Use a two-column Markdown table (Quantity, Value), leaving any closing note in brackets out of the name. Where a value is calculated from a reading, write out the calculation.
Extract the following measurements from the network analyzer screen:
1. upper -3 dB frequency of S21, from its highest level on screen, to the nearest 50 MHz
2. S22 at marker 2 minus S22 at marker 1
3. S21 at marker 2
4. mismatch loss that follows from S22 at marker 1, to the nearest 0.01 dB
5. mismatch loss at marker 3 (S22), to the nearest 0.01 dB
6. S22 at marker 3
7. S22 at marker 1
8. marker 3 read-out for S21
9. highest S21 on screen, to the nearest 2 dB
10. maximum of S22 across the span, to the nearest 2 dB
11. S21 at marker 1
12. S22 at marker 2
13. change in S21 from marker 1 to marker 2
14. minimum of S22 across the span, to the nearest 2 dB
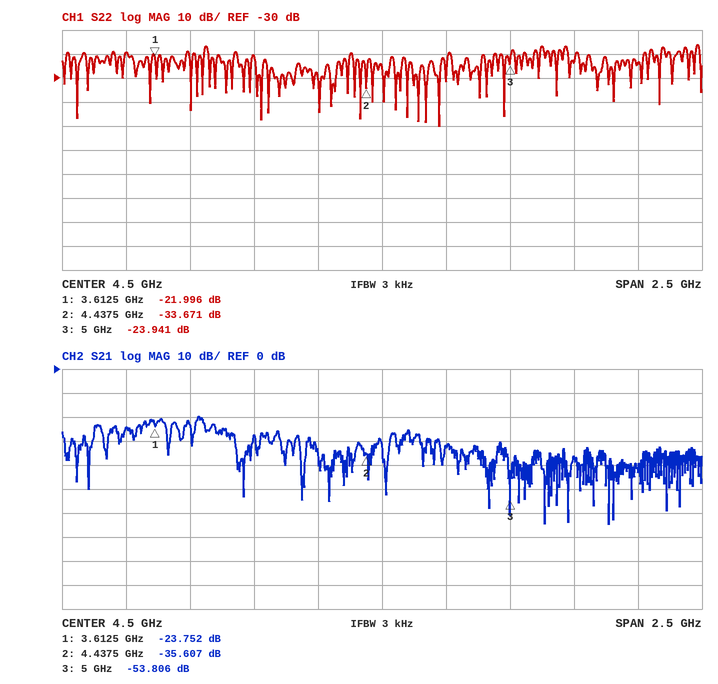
| Quantity | Value |
|---|---|
| upper -3 dB frequency of S21, from its highest level on screen, to the nearest 50 MHz | 3.80 GHz |
| S22 at marker 2 minus S22 at marker 1 | -33.671 − (-21.996) = -11.675 dB |
| S21 at marker 2 | -35.607 dB |
| mismatch loss that follows from S22 at marker 1, to the nearest 0.01 dB | −10 log10(1 − 10^(-21.996/10)) ≈ 0.03 dB |
| mismatch loss at marker 3 (S22), to the nearest 0.01 dB | −10 log10(1 − 10^(-23.941/10)) ≈ 0.02 dB |
| S22 at marker 3 | -23.941 dB |
| S22 at marker 1 | -21.996 dB |
| marker 3 read-out for S21 | -53.806 dB |
| highest S21 on screen, to the nearest 2 dB | -20 dB |
| maximum of S22 across the span, to the nearest 2 dB | -16 dB |
| S21 at marker 1 | -23.752 dB |
| S22 at marker 2 | -33.671 dB |
| change in S21 from marker 1 to marker 2 | -35.607 − (-23.752) = -11.855 dB |
| minimum of S22 across the span, to the nearest 2 dB | -50 dB |
